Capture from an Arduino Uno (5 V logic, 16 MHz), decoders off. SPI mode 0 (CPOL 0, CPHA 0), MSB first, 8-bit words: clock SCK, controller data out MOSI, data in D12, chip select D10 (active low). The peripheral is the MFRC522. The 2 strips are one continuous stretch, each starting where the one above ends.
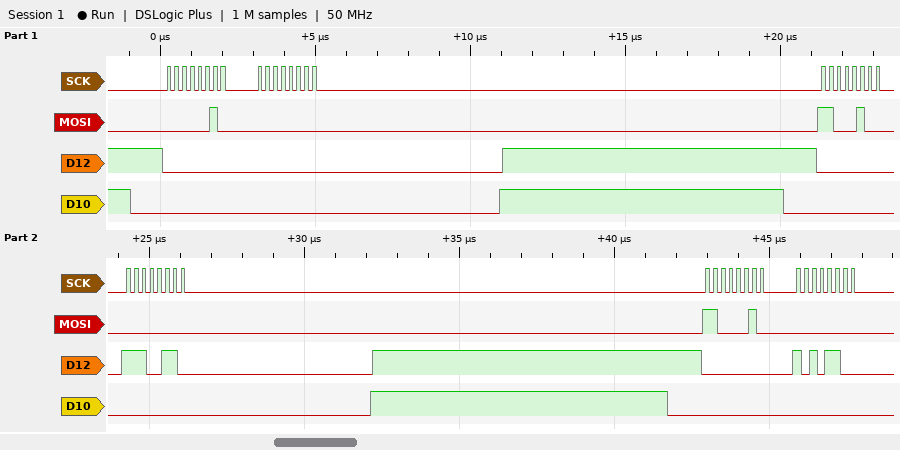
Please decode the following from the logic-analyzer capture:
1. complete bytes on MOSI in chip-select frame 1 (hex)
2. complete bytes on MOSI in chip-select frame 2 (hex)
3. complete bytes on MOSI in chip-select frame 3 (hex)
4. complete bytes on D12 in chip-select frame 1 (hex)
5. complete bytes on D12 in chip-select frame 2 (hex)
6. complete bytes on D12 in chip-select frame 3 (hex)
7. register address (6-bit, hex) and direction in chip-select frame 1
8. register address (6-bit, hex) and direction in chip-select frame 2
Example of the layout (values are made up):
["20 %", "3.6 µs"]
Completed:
["02 00", "C4 00", "C2 00", "00 00", "00 E6", "00 AC", "0x01 write", "0x22 read"]
